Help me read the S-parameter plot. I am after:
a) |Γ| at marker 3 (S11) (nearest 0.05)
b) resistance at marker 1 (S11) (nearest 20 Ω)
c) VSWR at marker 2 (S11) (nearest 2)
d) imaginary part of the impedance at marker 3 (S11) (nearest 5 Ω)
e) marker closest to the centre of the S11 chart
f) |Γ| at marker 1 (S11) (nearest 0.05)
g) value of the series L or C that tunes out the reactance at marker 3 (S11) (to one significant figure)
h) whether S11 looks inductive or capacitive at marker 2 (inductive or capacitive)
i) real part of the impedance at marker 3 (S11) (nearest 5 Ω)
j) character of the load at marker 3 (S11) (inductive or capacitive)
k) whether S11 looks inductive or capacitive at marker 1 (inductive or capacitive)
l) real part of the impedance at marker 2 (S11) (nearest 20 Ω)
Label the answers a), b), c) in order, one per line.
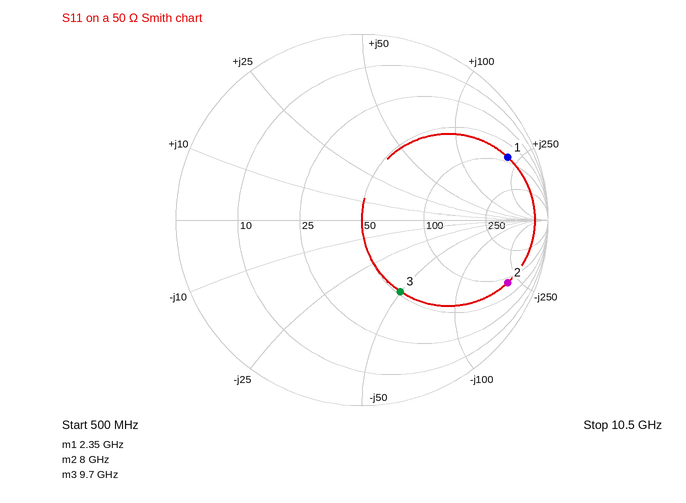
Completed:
a) 0.45
b) 80 Ω
c) 12
d) -50 Ω
e) marker 3
f) 0.85
g) 800 pH
h) capacitive
i) 50 Ω
j) capacitive
k) inductive
l) 80 Ω
